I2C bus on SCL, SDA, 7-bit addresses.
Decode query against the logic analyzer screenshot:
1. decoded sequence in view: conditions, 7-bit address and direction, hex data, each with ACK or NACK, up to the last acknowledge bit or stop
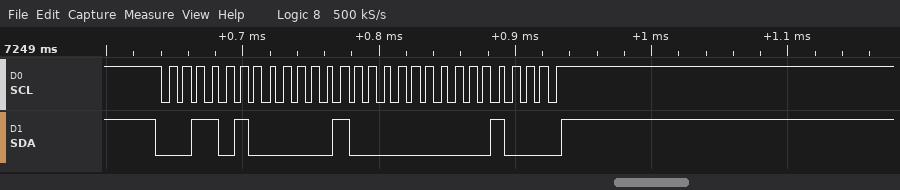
start, address 1A write ACK, 10 ACK, 04 ACK, stop
